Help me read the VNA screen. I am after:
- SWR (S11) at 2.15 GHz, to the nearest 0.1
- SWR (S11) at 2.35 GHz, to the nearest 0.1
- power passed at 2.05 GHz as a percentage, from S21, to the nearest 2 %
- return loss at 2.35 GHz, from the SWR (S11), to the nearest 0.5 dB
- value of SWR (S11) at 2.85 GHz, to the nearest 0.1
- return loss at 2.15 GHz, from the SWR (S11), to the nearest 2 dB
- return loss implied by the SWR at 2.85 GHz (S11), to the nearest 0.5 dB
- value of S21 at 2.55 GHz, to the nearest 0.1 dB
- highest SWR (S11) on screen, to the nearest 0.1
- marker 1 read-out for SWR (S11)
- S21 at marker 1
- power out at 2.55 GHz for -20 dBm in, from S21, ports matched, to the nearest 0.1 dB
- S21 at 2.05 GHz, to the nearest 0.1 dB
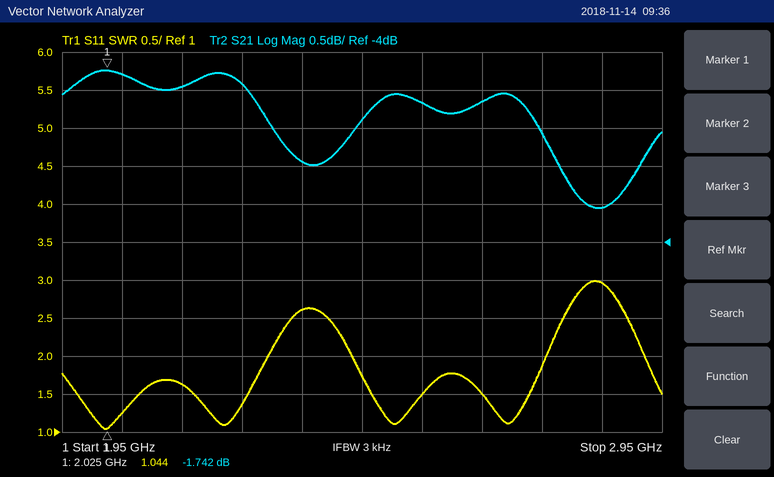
1.6
2.6
66 %
7.0 dB
3.0
12 dB
6.0 dB
-2.2 dB
3.0
1.044
-1.742 dB
-22.2 dBm
-1.8 dB
